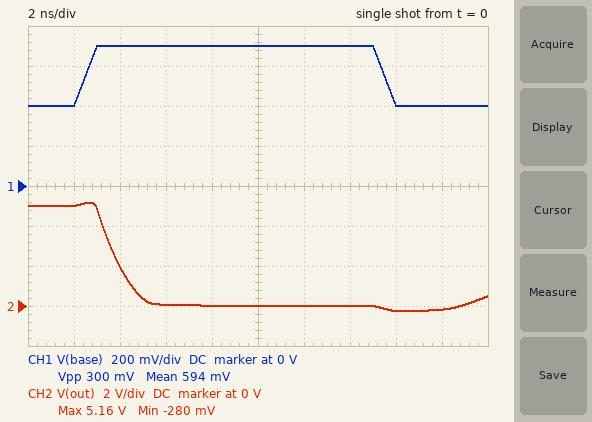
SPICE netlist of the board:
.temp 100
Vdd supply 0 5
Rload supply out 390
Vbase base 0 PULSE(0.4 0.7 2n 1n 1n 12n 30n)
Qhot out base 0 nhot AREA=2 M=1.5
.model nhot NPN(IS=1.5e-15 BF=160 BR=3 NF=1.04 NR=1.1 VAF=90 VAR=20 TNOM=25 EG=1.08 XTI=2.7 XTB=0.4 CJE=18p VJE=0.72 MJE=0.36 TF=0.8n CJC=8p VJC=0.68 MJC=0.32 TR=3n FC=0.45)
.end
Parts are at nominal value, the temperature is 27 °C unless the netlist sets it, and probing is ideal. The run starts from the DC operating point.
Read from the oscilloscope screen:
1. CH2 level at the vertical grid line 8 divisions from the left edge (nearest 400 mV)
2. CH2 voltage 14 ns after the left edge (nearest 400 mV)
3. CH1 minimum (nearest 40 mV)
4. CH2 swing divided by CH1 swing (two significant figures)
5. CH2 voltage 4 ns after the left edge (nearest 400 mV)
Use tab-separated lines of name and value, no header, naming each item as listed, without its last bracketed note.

CH2 level at the vertical grid line 8 divisions from the left edge	-400 mV
CH2 voltage 14 ns after the left edge	0 V
CH1 minimum	400 mV
CH2 swing divided by CH1 swing	18
CH2 voltage 4 ns after the left edge	2.0 V
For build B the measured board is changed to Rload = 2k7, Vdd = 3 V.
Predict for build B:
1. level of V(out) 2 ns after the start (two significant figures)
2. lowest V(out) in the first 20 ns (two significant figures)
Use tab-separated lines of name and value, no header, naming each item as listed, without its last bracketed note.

level of V(out) 2 ns after the start	3.0 V
lowest V(out) in the first 20 ns	-290 mV
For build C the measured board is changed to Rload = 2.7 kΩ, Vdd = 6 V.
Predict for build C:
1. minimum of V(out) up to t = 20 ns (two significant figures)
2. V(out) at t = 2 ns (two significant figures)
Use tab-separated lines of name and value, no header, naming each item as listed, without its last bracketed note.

minimum of V(out) up to t = 20 ns	-290 mV
V(out) at t = 2 ns	6.0 V
